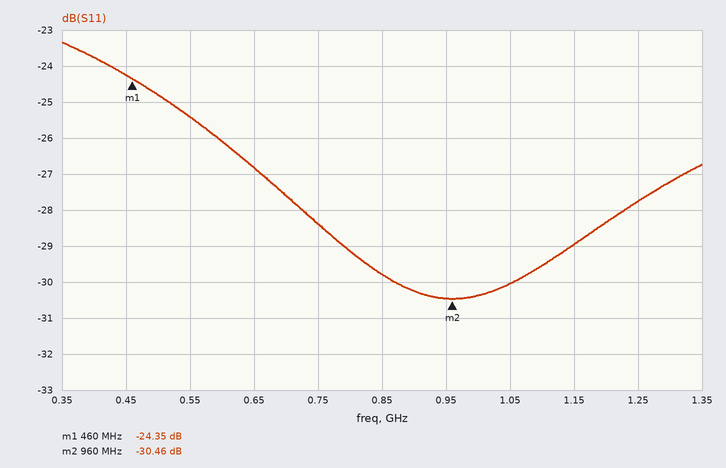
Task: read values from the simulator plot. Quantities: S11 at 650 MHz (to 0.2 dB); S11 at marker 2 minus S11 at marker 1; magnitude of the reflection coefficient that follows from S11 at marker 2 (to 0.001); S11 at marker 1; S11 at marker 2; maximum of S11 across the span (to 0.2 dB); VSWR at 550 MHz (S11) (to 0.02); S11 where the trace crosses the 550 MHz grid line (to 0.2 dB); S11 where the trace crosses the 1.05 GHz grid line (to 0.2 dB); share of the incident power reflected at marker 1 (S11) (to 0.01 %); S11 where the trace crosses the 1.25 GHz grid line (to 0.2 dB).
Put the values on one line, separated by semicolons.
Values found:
-26.8 dB; -6.11 dB; 0.030; -24.35 dB; -30.46 dB; -23.4 dB; 1.12; -25.4 dB; -30.0 dB; 0.37 %; -27.8 dB
